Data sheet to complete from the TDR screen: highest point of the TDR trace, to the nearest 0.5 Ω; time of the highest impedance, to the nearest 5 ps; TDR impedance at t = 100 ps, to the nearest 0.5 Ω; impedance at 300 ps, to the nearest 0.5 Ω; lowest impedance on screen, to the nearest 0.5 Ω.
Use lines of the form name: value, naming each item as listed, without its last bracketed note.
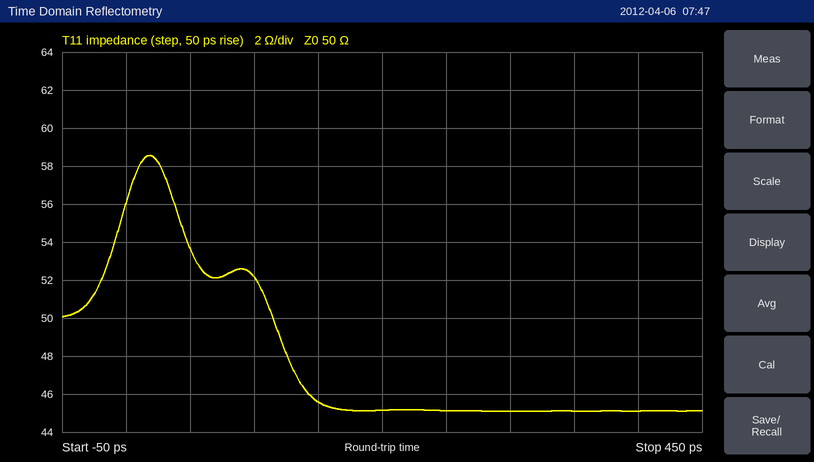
highest point of the TDR trace, to the nearest 0.5 Ω: 58.5 Ω
time of the highest impedance, to the nearest 5 ps: 20 ps
TDR impedance at t = 100 ps, to the nearest 0.5 Ω: 52.0 Ω
impedance at 300 ps, to the nearest 0.5 Ω: 45.0 Ω
lowest impedance on screen, to the nearest 0.5 Ω: 45.0 Ω
